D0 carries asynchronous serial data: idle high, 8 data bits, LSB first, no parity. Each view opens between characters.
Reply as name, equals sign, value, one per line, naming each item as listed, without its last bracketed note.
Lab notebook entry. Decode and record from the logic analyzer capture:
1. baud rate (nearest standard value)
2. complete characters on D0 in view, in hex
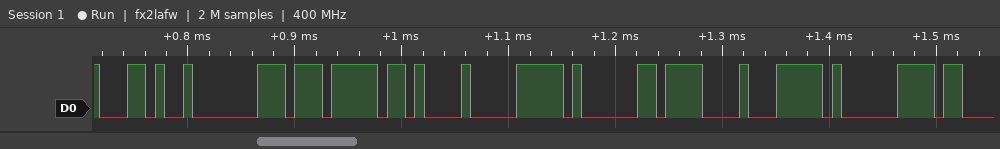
baud rate = 115200 baud
complete characters on D0 in view, in hex = 2C, C0, F7, 0B, F0, 81, 0F, 7C, E0
